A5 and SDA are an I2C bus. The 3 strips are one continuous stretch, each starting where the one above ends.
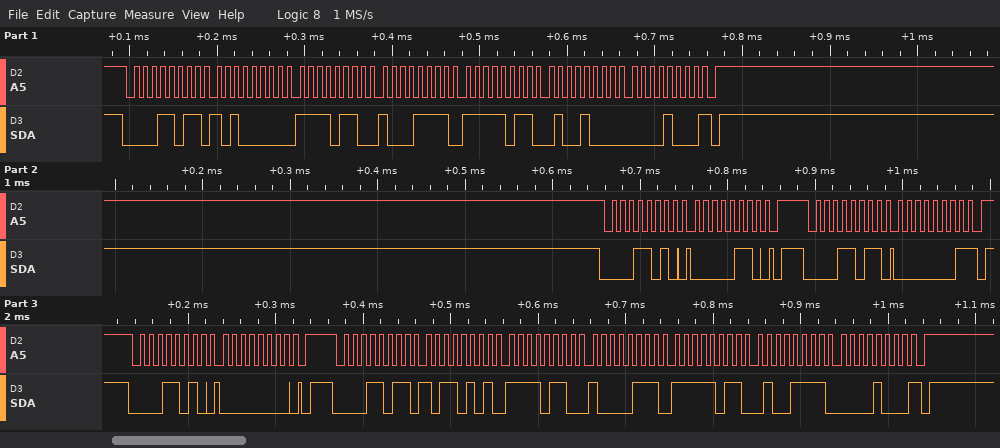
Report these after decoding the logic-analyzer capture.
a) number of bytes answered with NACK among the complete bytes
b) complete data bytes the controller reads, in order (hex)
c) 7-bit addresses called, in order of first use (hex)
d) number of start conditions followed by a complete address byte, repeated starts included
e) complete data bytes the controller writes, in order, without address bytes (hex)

3
A0 F6 8F FB 48 08 01 B5 F6 87 FB 4F 08
0x0D
5
06 00
